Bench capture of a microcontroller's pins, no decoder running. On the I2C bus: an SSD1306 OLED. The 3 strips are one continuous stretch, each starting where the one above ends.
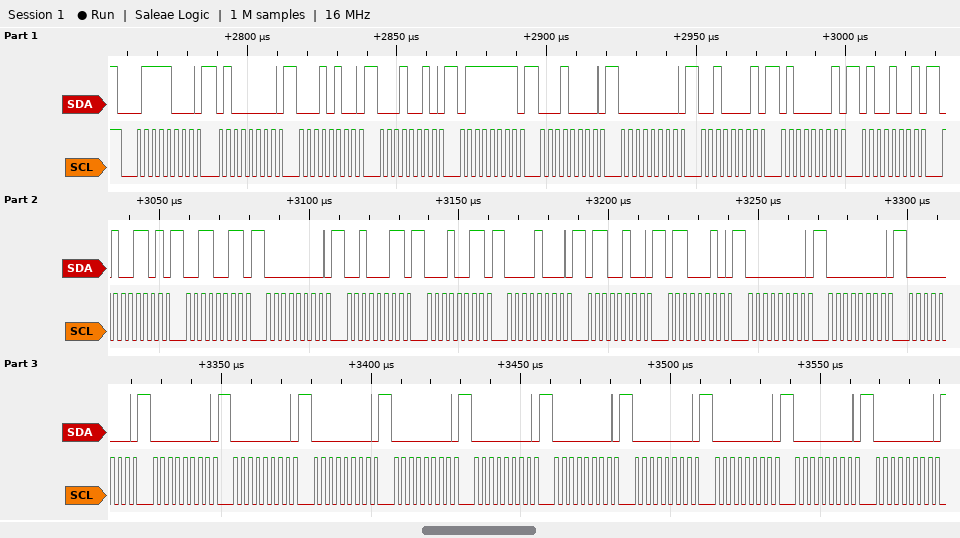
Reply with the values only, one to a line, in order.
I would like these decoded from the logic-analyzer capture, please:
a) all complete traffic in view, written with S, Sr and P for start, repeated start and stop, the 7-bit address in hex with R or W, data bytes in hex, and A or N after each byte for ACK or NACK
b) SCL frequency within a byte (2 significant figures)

S 3CW A 40 A 14 A 12 A 7F A 10 A 00 A 21 A 41 A 49 A 4D A 33 A 00 A 23 A 13 A 08 A 64 A 62 A 00 A 00 A 00 A 00 A 00 A 00 A 00 A 00 A 00 A 00 A 00 A 00 A 00 A
400 kHz
